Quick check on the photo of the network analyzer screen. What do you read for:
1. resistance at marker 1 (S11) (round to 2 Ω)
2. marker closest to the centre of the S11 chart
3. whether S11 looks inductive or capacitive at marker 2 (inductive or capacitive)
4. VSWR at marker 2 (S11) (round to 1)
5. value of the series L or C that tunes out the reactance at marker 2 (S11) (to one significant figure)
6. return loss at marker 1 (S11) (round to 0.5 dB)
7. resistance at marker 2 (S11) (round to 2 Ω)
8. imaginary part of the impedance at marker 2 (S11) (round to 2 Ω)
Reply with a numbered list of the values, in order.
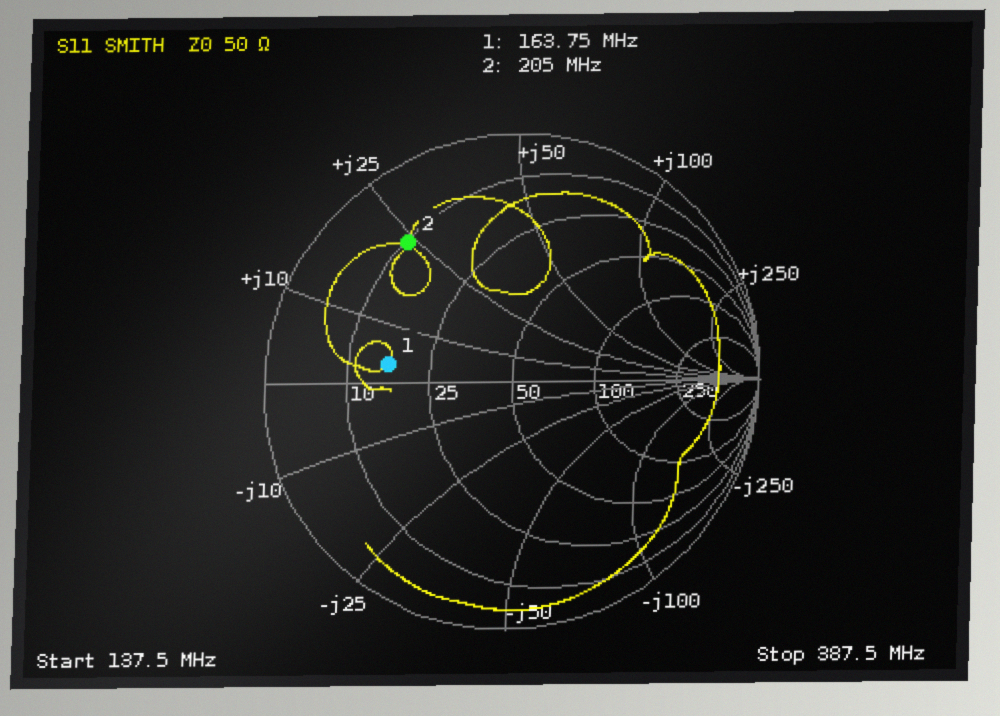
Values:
1. 16 Ω
2. marker 1
3. inductive
4. 6
5. 30 pF
6. 6.0 dB
7. 10 Ω
8. +24 Ω
